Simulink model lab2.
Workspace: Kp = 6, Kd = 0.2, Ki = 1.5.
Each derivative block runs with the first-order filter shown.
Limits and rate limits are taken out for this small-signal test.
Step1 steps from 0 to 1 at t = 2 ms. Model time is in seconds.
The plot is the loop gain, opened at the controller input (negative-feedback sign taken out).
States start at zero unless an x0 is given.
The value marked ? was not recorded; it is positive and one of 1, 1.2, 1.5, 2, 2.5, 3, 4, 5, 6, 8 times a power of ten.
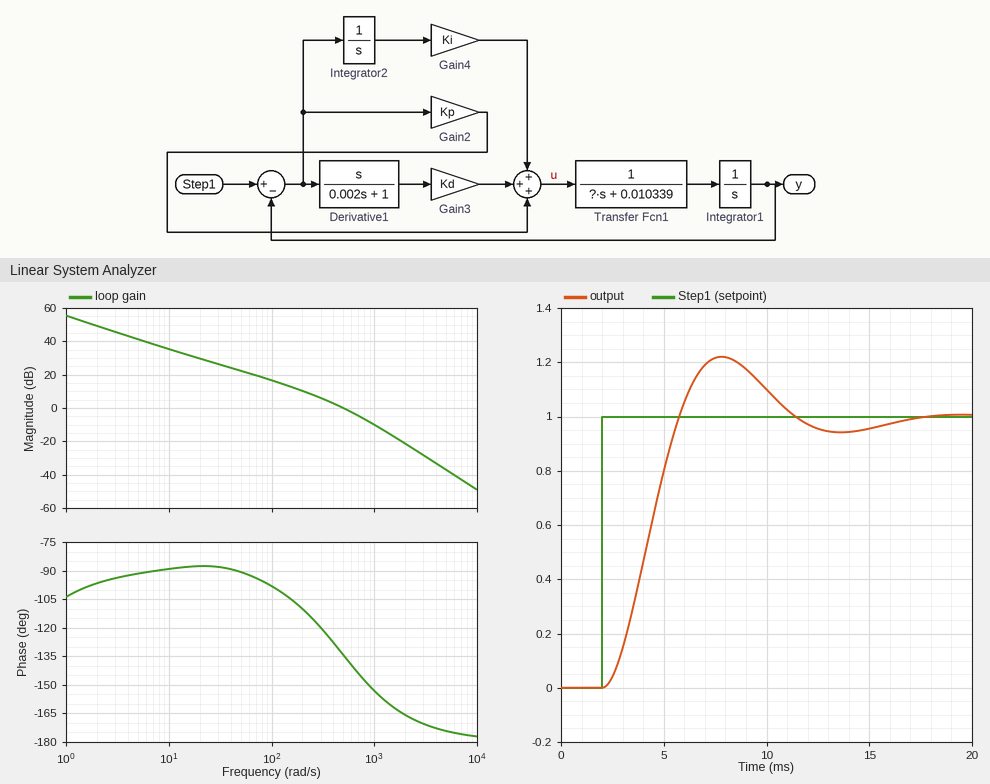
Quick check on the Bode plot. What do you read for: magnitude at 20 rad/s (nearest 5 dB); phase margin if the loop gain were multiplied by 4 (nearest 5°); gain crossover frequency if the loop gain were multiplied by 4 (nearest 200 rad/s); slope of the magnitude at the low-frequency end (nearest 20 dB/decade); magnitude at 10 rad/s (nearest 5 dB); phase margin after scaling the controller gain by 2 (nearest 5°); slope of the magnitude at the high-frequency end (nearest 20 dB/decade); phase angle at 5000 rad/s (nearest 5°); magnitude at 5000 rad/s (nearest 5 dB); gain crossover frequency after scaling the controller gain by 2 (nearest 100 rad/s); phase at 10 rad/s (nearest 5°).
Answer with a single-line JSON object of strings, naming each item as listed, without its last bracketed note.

{"magnitude at 20 rad/s": "30 dB", "phase margin if the loop gain were multiplied by 4": "25°", "gain crossover frequency if the loop gain were multiplied by 4": "1200 rad/s", "slope of the magnitude at the low-frequency end": "-20 dB/decade", "magnitude at 10 rad/s": "35 dB", "phase margin after scaling the controller gain by 2": "35°", "slope of the magnitude at the high-frequency end": "-40 dB/decade", "phase angle at 5000 rad/s": "-175°", "magnitude at 5000 rad/s": "-35 dB", "gain crossover frequency after scaling the controller gain by 2": "800 rad/s", "phase at 10 rad/s": "-90°"}
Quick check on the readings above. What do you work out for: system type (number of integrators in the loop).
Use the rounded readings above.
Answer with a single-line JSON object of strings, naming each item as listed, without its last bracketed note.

{"system type": "1"}
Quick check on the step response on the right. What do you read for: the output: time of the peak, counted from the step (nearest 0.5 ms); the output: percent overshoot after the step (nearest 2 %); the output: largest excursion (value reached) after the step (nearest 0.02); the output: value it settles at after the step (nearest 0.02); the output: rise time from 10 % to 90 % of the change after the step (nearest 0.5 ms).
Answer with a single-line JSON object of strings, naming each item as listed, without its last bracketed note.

{"the output: time of the peak, counted from the step": "6.0 ms", "the output: percent overshoot after the step": "22 %", "the output: largest excursion (value reached) after the step": "1.22", "the output: value it settles at after the step": "1.00", "the output: rise time from 10 % to 90 % of the change after the step": "2.5 ms"}
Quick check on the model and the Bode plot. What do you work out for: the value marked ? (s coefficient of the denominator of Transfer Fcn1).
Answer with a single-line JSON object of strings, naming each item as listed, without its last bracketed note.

{"the value marked ?": "0.0003"}
